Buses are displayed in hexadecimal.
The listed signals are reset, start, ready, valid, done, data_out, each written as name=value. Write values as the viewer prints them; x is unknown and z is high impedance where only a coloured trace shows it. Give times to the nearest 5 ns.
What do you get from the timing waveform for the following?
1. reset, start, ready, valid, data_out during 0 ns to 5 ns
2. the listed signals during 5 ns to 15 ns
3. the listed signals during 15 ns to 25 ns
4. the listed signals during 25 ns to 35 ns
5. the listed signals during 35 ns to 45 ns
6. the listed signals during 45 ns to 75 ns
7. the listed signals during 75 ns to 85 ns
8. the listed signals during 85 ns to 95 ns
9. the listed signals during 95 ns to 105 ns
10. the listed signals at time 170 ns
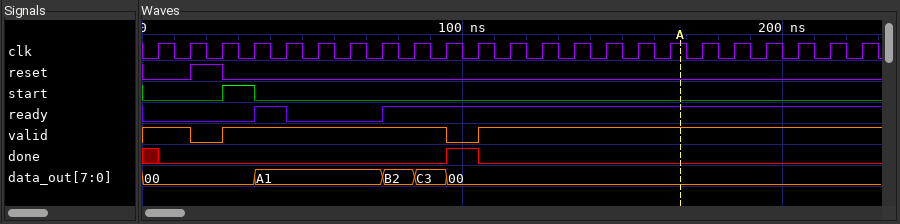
reset=0, start=0, ready=0, valid=1, data_out=00
reset=0, start=0, ready=0, valid=1, done=0, data_out=00
reset=1, start=0, ready=0, valid=0, done=0, data_out=00
reset=0, start=1, ready=0, valid=1, done=0, data_out=00
reset=0, start=0, ready=1, valid=1, done=0, data_out=A1
reset=0, start=0, ready=0, valid=1, done=0, data_out=A1
reset=0, start=0, ready=1, valid=1, done=0, data_out=B2
reset=0, start=0, ready=1, valid=1, done=0, data_out=C3
reset=0, start=0, ready=1, valid=0, done=1, data_out=00
reset=0, start=0, ready=1, valid=1, done=0, data_out=00
